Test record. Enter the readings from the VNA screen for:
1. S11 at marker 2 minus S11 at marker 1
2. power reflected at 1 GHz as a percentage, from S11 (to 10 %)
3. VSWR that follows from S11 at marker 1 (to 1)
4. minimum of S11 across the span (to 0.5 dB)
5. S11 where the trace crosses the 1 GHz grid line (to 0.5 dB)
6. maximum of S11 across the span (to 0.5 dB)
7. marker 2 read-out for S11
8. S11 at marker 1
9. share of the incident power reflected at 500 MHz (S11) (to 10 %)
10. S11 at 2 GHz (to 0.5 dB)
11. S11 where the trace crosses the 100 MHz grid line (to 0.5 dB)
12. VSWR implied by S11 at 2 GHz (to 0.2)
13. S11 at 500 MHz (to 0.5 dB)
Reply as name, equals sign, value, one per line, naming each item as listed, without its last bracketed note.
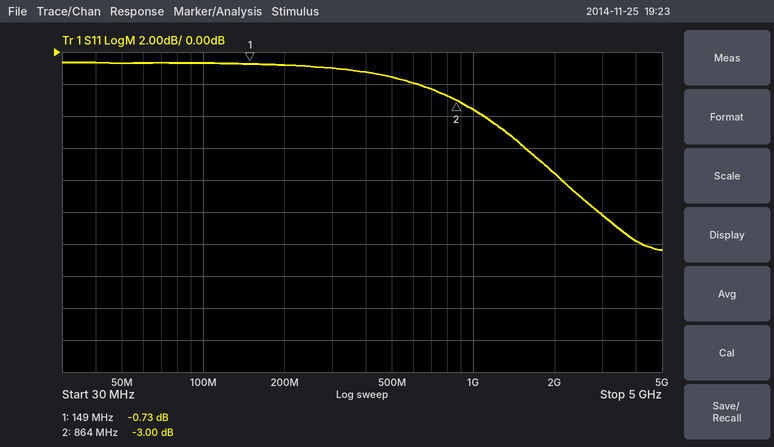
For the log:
S11 at marker 2 minus S11 at marker 1 = -2.27 dB
power reflected at 1 GHz as a percentage, from S11 = 40 %
VSWR that follows from S11 at marker 1 = 24
minimum of S11 across the span = -12.5 dB
S11 where the trace crosses the 1 GHz grid line = -3.5 dB
maximum of S11 across the span = -0.5 dB
marker 2 read-out for S11 = -3.00 dB
S11 at marker 1 = -0.73 dB
share of the incident power reflected at 500 MHz (S11) = 70 %
S11 at 2 GHz = -7.5 dB
S11 where the trace crosses the 100 MHz grid line = -0.5 dB
VSWR implied by S11 at 2 GHz = 2.4
S11 at 500 MHz = -1.5 dB
